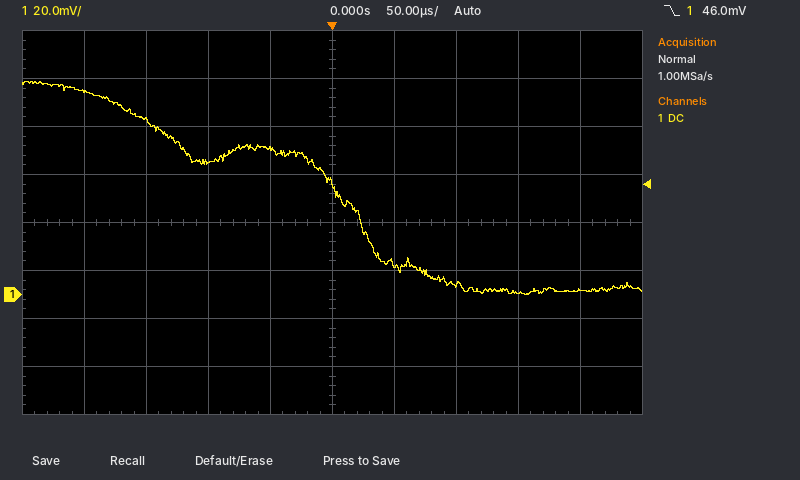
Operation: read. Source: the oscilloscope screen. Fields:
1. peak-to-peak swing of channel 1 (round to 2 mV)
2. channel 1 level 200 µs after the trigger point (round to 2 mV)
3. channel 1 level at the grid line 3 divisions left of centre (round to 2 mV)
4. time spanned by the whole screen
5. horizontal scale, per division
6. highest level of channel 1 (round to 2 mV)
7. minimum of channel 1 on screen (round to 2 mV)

88 mV
2 mV
72 mV
500 µs
50 µs
88 mV
0 mV
